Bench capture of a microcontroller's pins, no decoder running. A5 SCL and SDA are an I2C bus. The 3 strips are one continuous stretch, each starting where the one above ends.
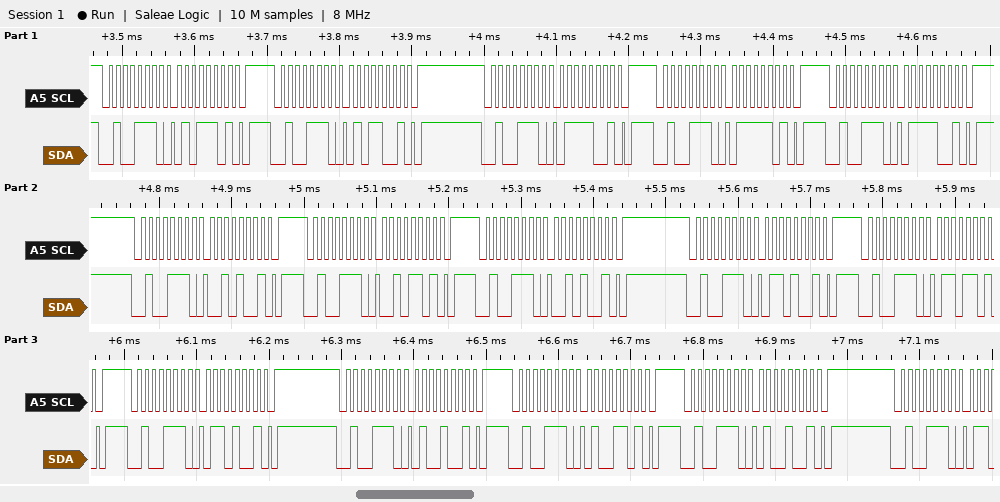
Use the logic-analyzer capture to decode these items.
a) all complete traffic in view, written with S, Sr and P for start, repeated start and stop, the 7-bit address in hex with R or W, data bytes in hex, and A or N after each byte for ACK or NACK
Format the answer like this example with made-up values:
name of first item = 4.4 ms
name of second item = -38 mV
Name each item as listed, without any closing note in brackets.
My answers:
all complete traffic in view, written with S, Sr and P for start, repeated start and stop, the 7-bit address in hex with R or W, data bytes in hex, and A or N after each byte for ACK or NACK = S 27W A 5D A P S 27W A 59 A P S 27W A 79 A P S 27W A 7D A P S 27W A 79 A P S 27W A 29 A P S 27W A 2D A P S 27W A 29 A P S 27W A 69 A P S 27W A 6D A P S 27W A 69 A P S 27W A 49 A P S 27W A 4D A P S 27W A 49 A P S 27W A
